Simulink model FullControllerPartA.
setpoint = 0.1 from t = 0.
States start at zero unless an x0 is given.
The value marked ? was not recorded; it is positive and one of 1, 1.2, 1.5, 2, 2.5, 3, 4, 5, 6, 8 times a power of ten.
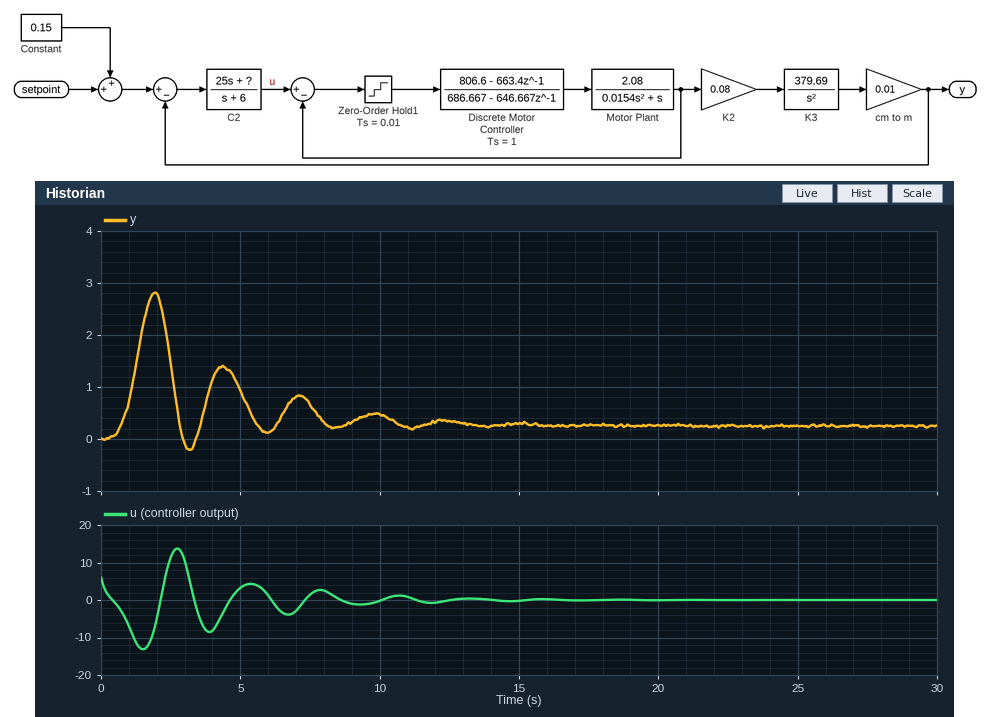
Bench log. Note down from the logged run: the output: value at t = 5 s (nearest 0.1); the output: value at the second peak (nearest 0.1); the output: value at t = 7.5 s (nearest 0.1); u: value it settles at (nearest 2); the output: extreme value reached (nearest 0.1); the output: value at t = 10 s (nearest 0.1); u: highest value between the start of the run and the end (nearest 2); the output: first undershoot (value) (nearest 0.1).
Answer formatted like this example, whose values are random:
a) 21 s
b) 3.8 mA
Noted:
a) 0.9
b) 1.4
c) 0.7
d) 0
e) 2.8
f) 0.5
g) 14
h) -0.2
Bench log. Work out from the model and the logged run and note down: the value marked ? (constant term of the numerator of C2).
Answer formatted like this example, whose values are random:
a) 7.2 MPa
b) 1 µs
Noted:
a) 6
